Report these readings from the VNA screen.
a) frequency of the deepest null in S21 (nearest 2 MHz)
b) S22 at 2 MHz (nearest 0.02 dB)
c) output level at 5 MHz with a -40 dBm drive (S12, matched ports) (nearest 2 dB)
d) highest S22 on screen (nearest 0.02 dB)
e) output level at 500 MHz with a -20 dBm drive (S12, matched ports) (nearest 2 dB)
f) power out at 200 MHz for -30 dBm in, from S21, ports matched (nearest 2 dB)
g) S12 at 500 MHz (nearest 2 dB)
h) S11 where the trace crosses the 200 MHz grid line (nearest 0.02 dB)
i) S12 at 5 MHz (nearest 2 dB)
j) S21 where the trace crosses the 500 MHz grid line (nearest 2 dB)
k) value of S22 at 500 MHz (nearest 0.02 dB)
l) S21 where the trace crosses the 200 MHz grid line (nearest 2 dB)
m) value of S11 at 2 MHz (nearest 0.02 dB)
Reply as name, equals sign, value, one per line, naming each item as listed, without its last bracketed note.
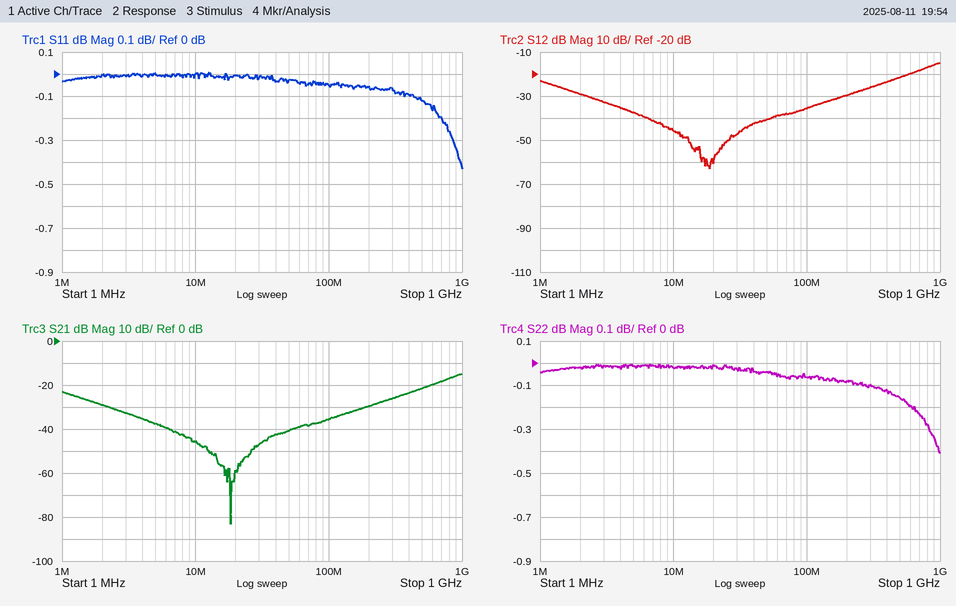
frequency of the deepest null in S21 = 18 MHz
S22 at 2 MHz = -0.02 dB
output level at 5 MHz with a -40 dBm drive (S12, matched ports) = -78 dBm
highest S22 on screen = 0.00 dB
output level at 500 MHz with a -20 dBm drive (S12, matched ports) = -42 dBm
power out at 200 MHz for -30 dBm in, from S21, ports matched = -60 dBm
S12 at 500 MHz = -22 dB
S11 where the trace crosses the 200 MHz grid line = -0.06 dB
S12 at 5 MHz = -38 dB
S21 where the trace crosses the 500 MHz grid line = -22 dB
value of S22 at 500 MHz = -0.16 dB
S21 where the trace crosses the 200 MHz grid line = -30 dB
value of S11 at 2 MHz = 0.00 dB
